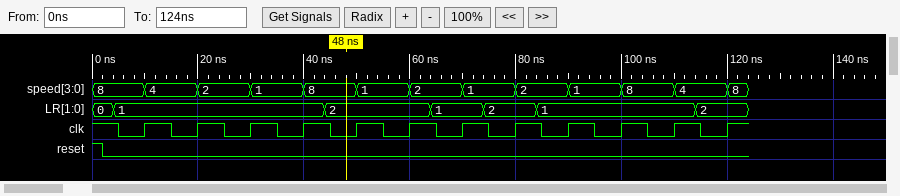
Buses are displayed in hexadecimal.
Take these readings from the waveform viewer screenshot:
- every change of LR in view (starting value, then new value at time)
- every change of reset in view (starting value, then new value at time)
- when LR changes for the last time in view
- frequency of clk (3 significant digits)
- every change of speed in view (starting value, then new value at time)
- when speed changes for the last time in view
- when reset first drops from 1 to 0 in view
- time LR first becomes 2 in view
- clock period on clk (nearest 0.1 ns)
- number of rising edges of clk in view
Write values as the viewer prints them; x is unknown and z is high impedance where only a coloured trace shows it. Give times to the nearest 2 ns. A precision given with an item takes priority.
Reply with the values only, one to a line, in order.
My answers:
0, 1 at 4 ns, 2 at 44 ns, 1 at 64 ns, 2 at 74 ns, 1 at 84 ns, 2 at 114 ns
1, 0 at 2 ns
114 ns
100 MHz
8, 4 at 10 ns, 2 at 20 ns, 1 at 30 ns, 8 at 40 ns, 1 at 50 ns, 2 at 60 ns, 1 at 70 ns, 2 at 80 ns, 1 at 90 ns, 8 at 100 ns, 4 at 110 ns, 8 at 120 ns
120 ns
2 ns
44 ns
10 ns
12
